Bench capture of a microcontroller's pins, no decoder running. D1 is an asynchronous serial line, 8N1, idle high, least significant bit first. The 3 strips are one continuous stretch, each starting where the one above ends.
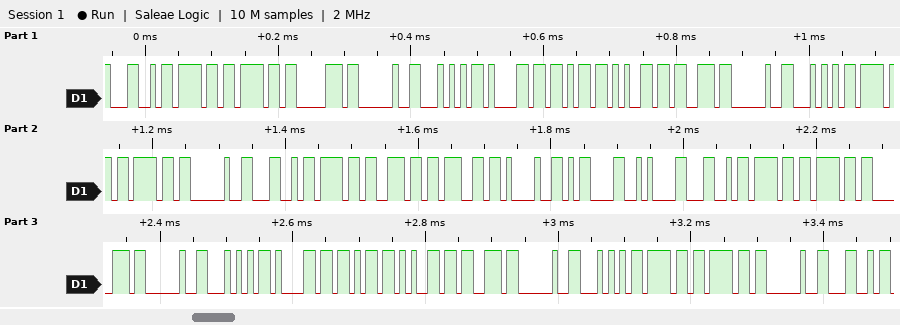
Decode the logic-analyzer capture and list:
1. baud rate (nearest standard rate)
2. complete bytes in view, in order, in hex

115200 baud
4C 6F 6F 70 20 54 61 6B 65 73 20 54 6F 6F 20 4C 6F 6E 67 21 0D 0A 4C 6F 6F 70 20 54 61 6B 65 73 20 54 6F 6F 20 4C
